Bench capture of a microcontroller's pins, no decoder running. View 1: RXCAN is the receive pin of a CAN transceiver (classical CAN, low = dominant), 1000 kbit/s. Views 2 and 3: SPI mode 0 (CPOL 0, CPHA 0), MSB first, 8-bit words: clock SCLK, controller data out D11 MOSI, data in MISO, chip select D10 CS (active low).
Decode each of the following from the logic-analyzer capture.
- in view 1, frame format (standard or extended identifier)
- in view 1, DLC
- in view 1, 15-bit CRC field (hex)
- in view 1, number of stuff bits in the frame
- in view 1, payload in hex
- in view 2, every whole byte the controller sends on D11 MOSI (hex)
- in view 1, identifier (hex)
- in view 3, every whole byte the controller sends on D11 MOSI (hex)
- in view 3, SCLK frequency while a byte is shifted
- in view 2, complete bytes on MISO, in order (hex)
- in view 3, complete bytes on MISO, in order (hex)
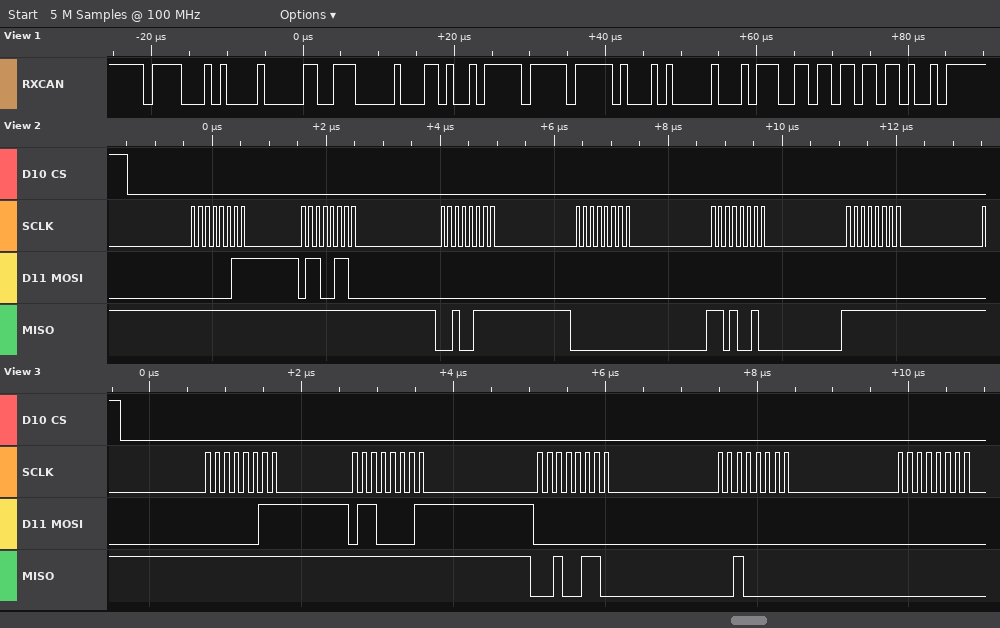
standard
8
0x6DB4
6
27 00 D2 FF FF 14 02 E6
03 66 00 00 00 00
0x78A
0x03 0x61 0x00 0x00 0x00
8 MHz
FF FF 27 00 D2 FF
0xFF 0xFF 0x26 0x20 0x00
